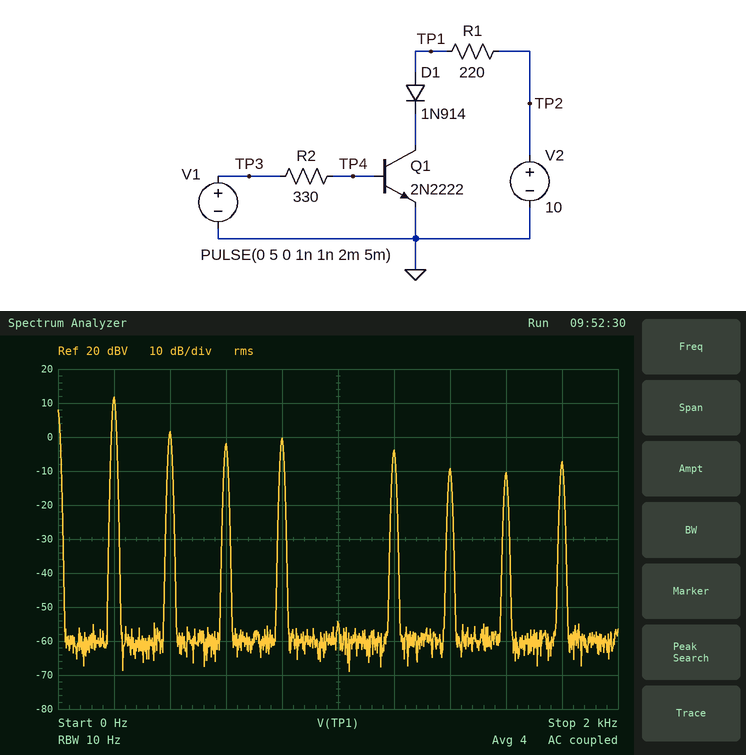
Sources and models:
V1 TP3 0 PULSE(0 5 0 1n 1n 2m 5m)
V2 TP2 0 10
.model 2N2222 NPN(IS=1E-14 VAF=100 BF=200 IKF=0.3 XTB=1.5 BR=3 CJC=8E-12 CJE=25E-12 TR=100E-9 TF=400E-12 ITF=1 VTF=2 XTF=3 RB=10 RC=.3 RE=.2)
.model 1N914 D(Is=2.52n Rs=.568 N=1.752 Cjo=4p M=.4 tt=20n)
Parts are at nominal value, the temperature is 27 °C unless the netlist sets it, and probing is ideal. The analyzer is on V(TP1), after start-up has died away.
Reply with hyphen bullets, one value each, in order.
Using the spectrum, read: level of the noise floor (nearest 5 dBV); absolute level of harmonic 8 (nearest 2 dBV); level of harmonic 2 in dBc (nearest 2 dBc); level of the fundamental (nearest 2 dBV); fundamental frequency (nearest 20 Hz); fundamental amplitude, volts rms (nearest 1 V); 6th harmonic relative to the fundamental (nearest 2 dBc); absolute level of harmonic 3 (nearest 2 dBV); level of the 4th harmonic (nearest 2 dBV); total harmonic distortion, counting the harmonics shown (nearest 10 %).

- -60 dBV
- -10 dBV
- -10 dBc
- 12 dBV
- 200 Hz
- 4 V
- -16 dBc
- -2 dBV
- 0 dBV
- 50 %
